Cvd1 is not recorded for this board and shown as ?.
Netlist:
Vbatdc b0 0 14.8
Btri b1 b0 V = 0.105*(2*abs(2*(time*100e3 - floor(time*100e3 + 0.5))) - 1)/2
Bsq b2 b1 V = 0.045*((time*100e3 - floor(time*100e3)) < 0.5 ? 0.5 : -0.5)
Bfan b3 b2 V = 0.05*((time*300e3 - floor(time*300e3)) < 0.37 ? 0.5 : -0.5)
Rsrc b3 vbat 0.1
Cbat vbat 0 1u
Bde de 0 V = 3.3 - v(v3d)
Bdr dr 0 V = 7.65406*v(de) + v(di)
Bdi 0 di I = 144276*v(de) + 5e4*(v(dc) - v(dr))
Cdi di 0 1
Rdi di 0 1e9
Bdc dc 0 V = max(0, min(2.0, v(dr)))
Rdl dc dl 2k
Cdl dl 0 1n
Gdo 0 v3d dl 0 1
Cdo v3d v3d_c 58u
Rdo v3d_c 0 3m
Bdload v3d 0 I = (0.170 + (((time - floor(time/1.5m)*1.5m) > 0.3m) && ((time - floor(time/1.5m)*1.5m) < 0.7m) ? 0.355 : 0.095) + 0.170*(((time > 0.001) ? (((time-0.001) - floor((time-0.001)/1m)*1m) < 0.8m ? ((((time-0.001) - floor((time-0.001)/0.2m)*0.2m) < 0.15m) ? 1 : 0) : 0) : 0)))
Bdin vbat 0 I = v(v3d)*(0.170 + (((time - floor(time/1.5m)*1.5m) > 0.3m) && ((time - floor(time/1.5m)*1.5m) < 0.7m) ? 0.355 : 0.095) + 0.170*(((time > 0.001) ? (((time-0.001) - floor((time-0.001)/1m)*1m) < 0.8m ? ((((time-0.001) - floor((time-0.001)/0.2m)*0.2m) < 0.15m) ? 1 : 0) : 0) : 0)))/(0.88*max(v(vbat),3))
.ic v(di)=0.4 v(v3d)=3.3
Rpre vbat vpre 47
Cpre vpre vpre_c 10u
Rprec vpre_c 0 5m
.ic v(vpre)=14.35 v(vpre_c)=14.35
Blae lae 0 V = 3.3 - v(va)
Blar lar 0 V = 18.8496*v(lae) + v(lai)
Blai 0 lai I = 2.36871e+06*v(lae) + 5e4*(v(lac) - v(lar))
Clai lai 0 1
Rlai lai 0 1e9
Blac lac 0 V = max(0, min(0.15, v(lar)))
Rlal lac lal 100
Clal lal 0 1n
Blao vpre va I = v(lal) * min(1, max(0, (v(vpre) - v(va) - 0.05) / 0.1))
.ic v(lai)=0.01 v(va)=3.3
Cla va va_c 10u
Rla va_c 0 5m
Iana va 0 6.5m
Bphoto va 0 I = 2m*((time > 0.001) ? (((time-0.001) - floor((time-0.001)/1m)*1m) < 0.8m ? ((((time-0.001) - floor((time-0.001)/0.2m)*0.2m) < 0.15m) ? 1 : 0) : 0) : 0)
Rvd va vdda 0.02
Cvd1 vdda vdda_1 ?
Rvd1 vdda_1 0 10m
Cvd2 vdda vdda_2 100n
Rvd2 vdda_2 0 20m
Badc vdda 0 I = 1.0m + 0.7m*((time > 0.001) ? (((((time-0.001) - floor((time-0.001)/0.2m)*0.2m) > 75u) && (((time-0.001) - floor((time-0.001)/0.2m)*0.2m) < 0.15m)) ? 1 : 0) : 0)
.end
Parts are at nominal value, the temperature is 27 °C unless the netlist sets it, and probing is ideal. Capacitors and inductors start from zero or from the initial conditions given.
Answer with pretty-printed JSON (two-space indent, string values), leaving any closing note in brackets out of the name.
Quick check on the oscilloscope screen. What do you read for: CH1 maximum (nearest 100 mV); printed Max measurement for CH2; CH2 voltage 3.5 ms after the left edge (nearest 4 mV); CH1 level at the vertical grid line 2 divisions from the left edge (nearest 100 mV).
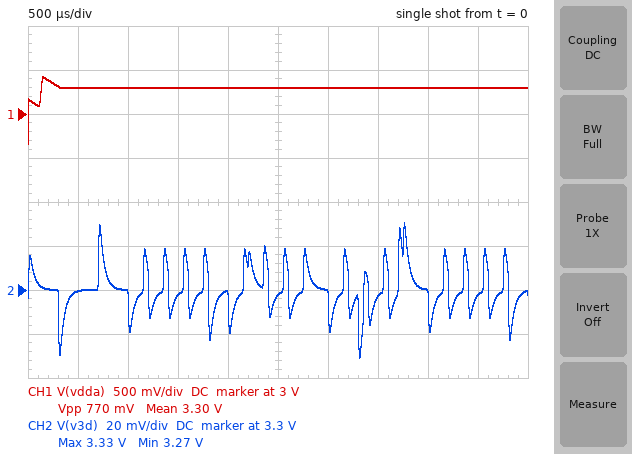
{
  "CH1 maximum": "3.4 V",
  "printed Max measurement for CH2": "3.33 V",
  "CH2 voltage 3.5 ms after the left edge": "3.296 V",
  "CH1 level at the vertical grid line 2 divisions from the left edge": "3.3 V"
}
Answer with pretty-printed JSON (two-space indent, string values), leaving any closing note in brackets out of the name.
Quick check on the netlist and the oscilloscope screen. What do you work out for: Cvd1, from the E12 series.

{
  "Cvd1, from the E12 series": "330 nF"
}
